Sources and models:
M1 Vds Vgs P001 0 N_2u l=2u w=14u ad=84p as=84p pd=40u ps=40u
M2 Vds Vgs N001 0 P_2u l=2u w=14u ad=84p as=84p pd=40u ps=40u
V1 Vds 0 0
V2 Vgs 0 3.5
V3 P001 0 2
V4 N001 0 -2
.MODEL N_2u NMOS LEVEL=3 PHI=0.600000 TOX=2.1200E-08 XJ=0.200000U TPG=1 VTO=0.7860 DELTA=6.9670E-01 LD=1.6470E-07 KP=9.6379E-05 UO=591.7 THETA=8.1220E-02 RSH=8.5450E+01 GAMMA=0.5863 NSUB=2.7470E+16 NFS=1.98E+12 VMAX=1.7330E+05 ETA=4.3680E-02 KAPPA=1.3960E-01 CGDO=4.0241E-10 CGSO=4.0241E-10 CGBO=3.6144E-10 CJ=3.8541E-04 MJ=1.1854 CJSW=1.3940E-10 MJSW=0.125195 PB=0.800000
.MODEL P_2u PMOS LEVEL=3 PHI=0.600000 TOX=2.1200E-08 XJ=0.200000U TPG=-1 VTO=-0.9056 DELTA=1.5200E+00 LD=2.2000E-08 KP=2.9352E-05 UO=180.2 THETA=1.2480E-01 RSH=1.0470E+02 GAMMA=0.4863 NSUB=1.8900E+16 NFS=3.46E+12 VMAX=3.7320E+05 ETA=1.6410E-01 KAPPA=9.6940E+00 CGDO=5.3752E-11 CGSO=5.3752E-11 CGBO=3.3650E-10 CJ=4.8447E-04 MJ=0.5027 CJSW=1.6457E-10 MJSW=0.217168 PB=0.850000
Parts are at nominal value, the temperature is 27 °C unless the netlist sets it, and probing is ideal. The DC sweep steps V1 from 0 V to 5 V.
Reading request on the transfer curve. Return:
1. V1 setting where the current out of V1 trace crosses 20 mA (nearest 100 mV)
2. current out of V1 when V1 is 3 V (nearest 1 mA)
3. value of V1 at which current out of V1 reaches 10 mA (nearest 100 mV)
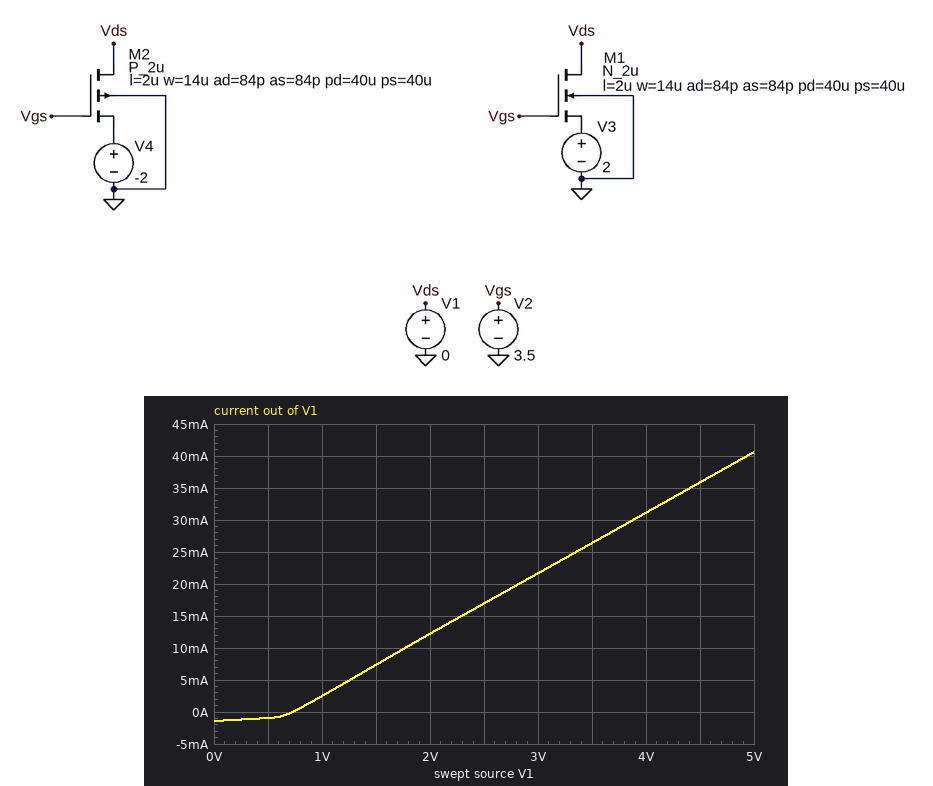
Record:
2.8 V
22 mA
1.8 V
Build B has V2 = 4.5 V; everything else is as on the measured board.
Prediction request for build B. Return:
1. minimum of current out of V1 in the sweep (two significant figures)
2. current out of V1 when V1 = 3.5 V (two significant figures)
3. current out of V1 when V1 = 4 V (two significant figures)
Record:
-2.1 mA
27 mA
32 mA
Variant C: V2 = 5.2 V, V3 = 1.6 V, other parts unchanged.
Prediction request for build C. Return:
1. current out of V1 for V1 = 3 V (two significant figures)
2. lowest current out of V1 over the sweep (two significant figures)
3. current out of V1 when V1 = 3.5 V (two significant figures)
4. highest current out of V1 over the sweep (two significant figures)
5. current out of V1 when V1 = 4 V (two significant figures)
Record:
23 mA
-2.2 mA
28 mA
42 mA
32 mA
